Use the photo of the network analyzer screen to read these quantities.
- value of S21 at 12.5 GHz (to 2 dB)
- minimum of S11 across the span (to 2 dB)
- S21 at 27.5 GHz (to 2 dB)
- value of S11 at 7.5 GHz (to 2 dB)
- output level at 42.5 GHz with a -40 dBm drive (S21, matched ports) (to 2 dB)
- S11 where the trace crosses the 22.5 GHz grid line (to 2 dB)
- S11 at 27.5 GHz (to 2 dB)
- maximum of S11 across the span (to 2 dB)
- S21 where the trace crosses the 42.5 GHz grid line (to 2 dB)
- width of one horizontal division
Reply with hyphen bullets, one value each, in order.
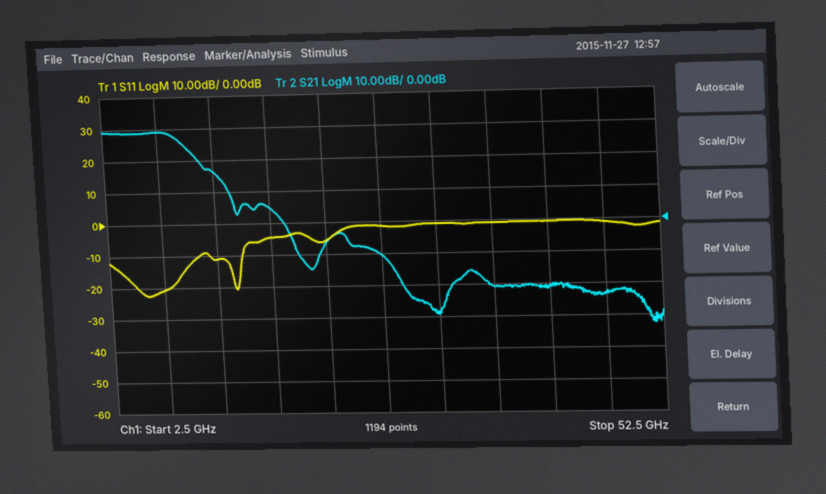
- 16 dB
- -22 dB
- -10 dB
- -20 dB
- -60 dBm
- -6 dB
- -2 dB
- 0 dB
- -20 dB
- 5 GHz
